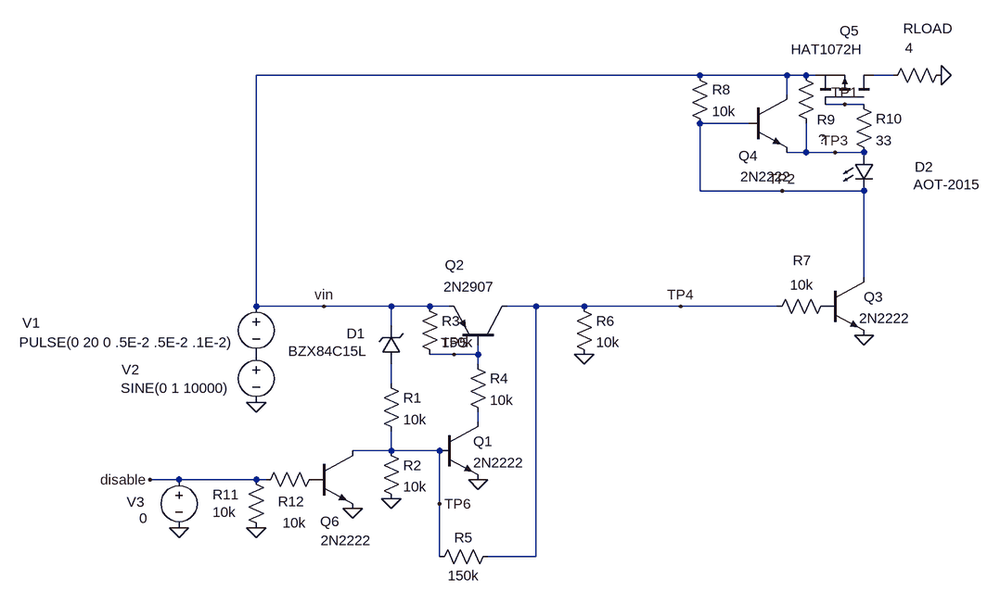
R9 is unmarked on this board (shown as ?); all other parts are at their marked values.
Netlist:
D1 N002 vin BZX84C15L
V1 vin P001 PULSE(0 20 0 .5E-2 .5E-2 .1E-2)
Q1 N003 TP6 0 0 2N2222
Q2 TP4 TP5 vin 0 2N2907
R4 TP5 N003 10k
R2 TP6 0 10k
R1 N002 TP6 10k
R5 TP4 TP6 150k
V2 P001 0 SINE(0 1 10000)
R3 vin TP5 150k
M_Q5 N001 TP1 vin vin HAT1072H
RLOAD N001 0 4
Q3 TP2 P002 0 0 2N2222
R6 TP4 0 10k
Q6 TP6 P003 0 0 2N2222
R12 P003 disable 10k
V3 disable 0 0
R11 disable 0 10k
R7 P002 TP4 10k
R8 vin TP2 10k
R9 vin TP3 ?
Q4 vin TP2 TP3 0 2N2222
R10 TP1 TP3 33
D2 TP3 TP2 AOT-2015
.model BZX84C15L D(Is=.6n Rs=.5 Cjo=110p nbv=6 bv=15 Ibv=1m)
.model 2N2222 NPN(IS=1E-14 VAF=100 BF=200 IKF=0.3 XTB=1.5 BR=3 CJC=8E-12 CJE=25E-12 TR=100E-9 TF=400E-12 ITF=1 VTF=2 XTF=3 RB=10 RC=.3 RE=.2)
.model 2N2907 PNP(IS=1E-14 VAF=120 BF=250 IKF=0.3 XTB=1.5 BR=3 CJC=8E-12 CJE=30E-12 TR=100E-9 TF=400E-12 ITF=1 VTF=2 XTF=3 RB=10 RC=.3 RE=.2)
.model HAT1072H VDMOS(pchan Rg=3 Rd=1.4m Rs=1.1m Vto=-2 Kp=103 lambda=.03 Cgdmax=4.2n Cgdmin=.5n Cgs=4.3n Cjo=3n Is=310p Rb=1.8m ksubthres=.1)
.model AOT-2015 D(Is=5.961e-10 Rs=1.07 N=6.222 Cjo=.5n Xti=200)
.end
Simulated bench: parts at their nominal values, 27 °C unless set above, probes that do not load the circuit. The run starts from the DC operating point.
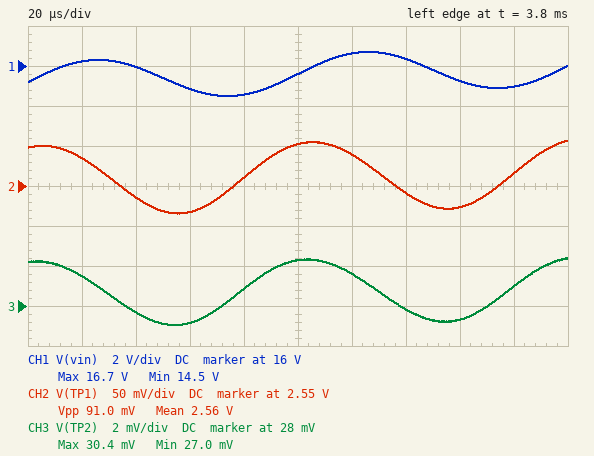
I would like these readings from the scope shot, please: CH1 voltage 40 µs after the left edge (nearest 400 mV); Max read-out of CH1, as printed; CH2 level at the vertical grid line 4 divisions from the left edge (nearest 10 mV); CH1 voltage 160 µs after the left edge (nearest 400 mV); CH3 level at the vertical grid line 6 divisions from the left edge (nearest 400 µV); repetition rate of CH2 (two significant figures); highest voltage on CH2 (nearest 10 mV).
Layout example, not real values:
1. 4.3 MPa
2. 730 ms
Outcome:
1. 16.0 V
2. 16.7 V
3. 2.56 V
4. 15.2 V
5. 29.6 mV
6. 10 kHz
7. 2.61 V
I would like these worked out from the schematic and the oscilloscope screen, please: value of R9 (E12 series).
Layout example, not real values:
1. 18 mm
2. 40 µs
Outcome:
1. 3.3 kΩ
